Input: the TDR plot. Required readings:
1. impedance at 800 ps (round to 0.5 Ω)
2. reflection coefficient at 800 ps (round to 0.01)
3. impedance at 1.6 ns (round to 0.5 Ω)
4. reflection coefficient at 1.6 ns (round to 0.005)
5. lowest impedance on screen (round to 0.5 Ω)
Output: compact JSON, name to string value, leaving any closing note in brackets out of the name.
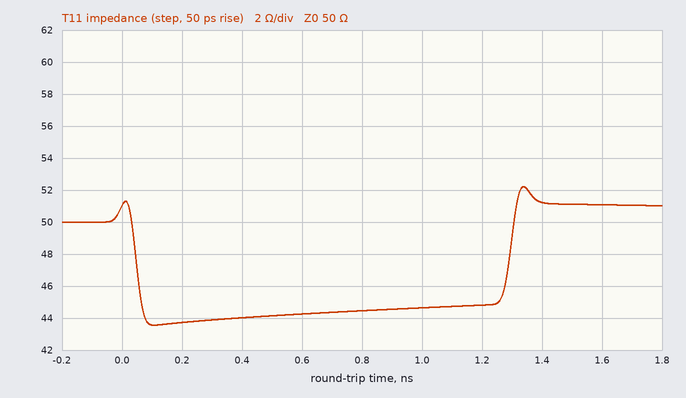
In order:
{"impedance at 800 ps": "44.5 Ω", "reflection coefficient at 800 ps": "-0.06", "impedance at 1.6 ns": "51.0 Ω", "reflection coefficient at 1.6 ns": "+0.010", "lowest impedance on screen": "43.5 Ω"}
